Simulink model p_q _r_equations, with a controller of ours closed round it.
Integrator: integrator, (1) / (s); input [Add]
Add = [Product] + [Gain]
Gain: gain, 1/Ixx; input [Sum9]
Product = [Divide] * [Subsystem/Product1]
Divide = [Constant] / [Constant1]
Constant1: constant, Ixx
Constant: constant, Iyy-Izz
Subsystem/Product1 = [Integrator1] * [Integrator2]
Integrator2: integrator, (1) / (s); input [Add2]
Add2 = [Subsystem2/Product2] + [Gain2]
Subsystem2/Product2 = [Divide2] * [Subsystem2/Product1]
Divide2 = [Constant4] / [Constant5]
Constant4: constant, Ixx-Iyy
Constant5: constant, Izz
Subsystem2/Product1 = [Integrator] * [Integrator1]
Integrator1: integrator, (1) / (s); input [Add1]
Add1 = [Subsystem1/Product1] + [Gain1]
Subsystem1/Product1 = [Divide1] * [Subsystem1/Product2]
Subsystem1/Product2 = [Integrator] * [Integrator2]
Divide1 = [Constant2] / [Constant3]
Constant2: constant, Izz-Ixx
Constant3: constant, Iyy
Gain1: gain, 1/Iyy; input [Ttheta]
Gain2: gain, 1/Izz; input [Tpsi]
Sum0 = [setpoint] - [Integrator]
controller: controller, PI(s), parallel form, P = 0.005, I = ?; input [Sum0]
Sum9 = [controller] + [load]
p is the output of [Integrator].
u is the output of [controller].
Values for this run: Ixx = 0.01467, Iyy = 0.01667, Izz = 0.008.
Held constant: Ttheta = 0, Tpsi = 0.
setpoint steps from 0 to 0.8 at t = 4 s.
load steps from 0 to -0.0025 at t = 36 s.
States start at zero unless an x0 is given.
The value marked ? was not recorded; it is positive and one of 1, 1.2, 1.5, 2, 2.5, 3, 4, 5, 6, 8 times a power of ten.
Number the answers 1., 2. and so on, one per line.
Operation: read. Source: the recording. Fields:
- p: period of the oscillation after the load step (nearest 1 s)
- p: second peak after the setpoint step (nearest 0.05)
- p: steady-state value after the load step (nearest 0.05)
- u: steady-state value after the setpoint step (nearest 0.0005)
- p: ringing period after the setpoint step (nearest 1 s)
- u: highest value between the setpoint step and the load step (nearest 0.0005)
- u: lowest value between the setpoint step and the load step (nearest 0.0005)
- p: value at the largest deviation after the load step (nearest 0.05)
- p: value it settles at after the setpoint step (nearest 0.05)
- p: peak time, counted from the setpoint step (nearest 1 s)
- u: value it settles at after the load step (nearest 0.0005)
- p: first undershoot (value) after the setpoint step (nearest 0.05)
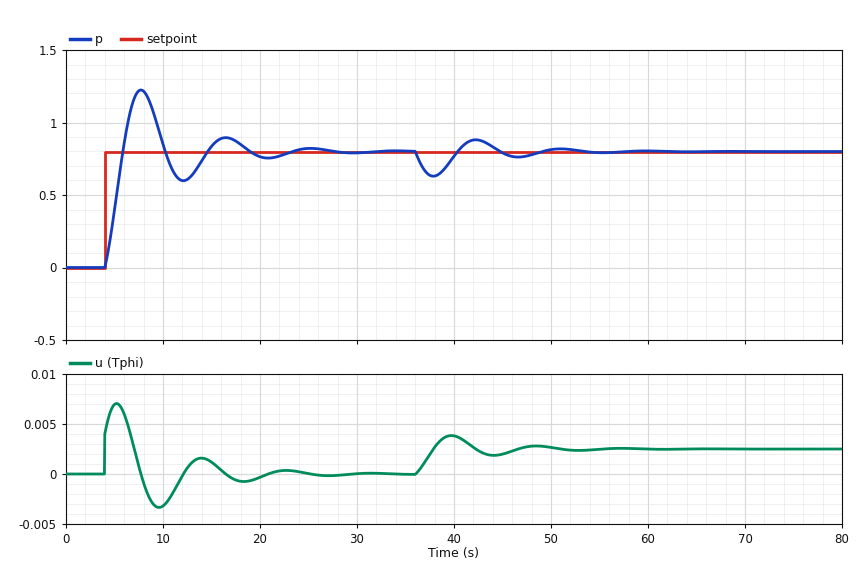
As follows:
1. 9 s
2. 0.90
3. 0.80
4. 0.0000
5. 9 s
6. 0.0070
7. -0.0035
8. 0.65
9. 0.80
10. 4 s
11. 0.0025
12. 0.60
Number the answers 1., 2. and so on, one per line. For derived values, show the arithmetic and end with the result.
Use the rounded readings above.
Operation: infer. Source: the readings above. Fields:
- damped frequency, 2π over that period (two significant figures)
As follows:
1. 2π / 9 = 0.70 rad/s
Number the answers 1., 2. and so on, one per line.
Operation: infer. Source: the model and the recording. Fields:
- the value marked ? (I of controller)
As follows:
1. 0.008
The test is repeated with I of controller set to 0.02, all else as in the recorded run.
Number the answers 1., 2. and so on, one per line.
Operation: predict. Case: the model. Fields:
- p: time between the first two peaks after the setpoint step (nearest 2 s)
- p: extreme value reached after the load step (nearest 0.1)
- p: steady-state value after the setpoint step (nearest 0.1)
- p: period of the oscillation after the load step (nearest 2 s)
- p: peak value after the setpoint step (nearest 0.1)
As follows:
1. 6 s
2. 0.7
3. 0.8
4. 6 s
5. 1.3
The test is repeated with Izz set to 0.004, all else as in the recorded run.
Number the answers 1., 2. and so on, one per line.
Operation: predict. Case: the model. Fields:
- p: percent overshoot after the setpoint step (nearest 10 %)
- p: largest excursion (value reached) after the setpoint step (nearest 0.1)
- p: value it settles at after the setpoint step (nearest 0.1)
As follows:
1. 50 %
2. 1.2
3. 0.8
